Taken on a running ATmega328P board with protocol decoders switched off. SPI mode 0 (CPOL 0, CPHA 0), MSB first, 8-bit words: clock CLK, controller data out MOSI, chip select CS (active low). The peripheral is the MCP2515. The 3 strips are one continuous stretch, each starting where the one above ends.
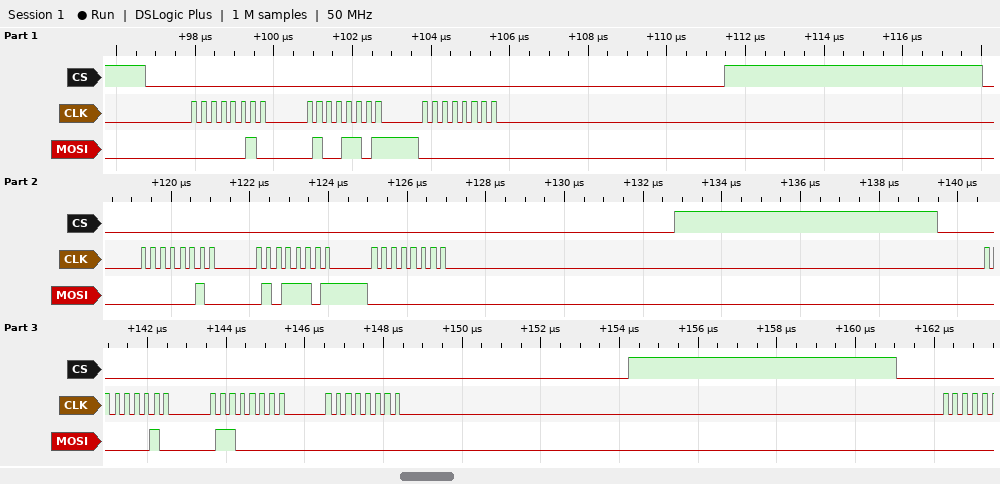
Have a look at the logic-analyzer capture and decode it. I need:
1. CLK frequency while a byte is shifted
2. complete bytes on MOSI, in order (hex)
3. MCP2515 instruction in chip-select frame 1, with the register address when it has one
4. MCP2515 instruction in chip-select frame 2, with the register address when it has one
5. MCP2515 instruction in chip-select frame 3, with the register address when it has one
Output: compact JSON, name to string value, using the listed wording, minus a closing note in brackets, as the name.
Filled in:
{"CLK frequency while a byte is shifted": "4 MHz", "complete bytes on MOSI, in order": "0x02 0x4D 0x00 0x02 0x5D 0x00 0x02 0x60 0x00", "MCP2515 instruction in chip-select frame 1, with the register address when it has one": "WRITE 0x4D", "MCP2515 instruction in chip-select frame 2, with the register address when it has one": "WRITE 0x5D", "MCP2515 instruction in chip-select frame 3, with the register address when it has one": "WRITE 0x60"}
